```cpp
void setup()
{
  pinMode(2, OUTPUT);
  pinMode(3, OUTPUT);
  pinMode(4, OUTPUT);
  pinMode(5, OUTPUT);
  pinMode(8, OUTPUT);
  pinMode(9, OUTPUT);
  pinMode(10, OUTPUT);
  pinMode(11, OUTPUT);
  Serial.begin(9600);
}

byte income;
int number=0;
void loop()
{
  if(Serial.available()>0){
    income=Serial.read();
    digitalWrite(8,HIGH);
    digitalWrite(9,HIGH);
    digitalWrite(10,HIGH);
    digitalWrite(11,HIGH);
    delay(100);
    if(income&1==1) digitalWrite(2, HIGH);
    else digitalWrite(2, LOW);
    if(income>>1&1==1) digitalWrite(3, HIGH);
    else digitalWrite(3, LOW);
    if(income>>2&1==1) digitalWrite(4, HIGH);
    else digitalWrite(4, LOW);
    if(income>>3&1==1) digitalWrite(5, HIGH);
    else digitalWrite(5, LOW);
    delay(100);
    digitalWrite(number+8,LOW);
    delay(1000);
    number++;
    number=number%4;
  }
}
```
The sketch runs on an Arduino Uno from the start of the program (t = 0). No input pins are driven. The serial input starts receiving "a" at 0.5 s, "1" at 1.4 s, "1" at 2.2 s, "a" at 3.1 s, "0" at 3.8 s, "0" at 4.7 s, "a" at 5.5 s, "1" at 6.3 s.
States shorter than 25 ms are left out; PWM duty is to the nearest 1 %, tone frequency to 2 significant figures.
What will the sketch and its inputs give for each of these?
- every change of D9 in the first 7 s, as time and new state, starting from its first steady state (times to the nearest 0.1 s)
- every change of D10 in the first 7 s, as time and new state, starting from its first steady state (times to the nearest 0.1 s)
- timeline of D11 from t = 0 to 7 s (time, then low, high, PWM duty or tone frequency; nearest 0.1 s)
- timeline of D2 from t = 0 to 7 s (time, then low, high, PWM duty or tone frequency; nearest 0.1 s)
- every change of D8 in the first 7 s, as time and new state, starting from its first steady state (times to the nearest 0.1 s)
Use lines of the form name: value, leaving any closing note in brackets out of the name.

every change of D9 in the first 7 s, as time and new state, starting from its first steady state: 0 s low; 0.5 s high; 1.9 s low; 2.9 s high; 6.7 s low
every change of D10 in the first 7 s, as time and new state, starting from its first steady state: 0 s low; 0.5 s high; 3.1 s low; 4.1 s high
timeline of D11 from t = 0 to 7 s: 0 s low; 0.5 s high; 4.3 s low; 5.3 s high
timeline of D2 from t = 0 to 7 s: 0 s low; 0.6 s high; 5.4 s low
every change of D8 in the first 7 s, as time and new state, starting from its first steady state: 0 s low; 0.5 s high; 0.7 s low; 1.7 s high; 5.5 s low; 6.5 s high
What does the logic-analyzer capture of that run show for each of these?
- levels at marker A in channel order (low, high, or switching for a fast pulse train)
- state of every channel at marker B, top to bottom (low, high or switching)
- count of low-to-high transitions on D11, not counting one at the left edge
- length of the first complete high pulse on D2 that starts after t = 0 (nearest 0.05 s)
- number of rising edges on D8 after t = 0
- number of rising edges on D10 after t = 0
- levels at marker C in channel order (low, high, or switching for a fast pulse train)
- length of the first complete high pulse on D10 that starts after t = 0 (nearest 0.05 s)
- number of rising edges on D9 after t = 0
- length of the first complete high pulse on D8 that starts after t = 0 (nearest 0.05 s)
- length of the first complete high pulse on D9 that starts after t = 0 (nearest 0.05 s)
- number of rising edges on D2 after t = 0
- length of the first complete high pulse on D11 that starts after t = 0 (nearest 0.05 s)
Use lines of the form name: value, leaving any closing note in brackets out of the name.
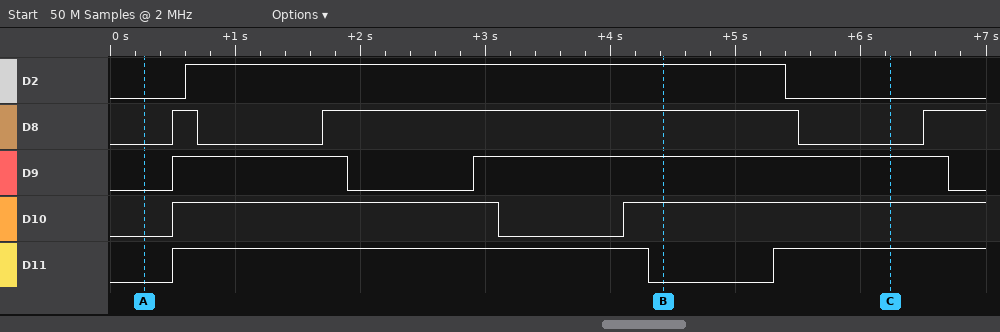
levels at marker A in channel order: D2 low, D8 low, D9 low, D10 low, D11 low
state of every channel at marker B, top to bottom: D2 high, D8 high, D9 high, D10 high, D11 low
count of low-to-high transitions on D11, not counting one at the left edge: 2
length of the first complete high pulse on D2 that starts after t = 0: 4.80 s
number of rising edges on D8 after t = 0: 3
number of rising edges on D10 after t = 0: 2
levels at marker C in channel order: D2 low, D8 low, D9 high, D10 high, D11 high
length of the first complete high pulse on D10 that starts after t = 0: 2.60 s
number of rising edges on D9 after t = 0: 2
length of the first complete high pulse on D8 that starts after t = 0: 0.20 s
length of the first complete high pulse on D9 that starts after t = 0: 1.40 s
number of rising edges on D2 after t = 0: 1
length of the first complete high pulse on D11 that starts after t = 0: 3.80 s
